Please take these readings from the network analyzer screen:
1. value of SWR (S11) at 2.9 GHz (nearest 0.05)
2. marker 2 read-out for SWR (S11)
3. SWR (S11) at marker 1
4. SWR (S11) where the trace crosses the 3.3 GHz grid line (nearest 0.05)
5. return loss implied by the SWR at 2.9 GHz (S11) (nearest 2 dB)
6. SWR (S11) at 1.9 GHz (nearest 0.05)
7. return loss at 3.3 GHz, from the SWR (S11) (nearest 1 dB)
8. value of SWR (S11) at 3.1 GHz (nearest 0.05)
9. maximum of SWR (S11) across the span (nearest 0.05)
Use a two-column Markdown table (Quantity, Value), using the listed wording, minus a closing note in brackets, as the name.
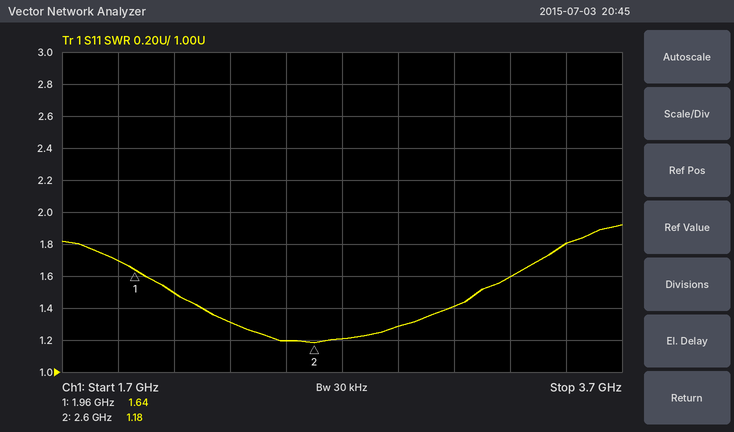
| Quantity | Value |
|---|---|
| value of SWR (S11) at 2.9 GHz | 1.30 |
| marker 2 read-out for SWR | 1.18 |
| SWR (S11) at marker 1 | 1.64 |
| SWR (S11) where the trace crosses the 3.3 GHz grid line | 1.60 |
| return loss implied by the SWR at 2.9 GHz (S11) | 18 dB |
| SWR (S11) at 1.9 GHz | 1.70 |
| return loss at 3.3 GHz, from the SWR (S11) | 13 dB |
| value of SWR (S11) at 3.1 GHz | 1.40 |
| maximum of SWR (S11) across the span | 1.90 |
